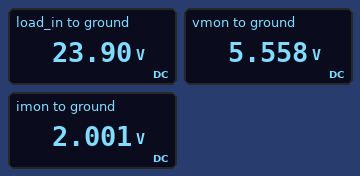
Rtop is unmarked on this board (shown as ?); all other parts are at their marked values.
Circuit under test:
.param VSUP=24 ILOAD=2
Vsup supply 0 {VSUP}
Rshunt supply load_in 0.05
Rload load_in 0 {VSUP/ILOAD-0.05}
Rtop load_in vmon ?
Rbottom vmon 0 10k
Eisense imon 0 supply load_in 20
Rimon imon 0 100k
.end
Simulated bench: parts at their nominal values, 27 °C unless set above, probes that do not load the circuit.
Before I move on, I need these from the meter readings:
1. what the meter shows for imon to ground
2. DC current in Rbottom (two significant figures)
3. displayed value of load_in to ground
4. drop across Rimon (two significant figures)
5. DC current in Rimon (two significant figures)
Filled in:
2.001 V
560 µA
23.90 V
2.0 V
20 µA
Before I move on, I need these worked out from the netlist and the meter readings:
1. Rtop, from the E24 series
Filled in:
33 kΩ
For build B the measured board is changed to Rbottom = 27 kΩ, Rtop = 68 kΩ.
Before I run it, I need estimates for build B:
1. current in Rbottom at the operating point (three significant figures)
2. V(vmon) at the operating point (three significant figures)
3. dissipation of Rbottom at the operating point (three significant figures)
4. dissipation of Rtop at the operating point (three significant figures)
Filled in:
252 µA
6.79 V
1.71 mW
4.30 mW
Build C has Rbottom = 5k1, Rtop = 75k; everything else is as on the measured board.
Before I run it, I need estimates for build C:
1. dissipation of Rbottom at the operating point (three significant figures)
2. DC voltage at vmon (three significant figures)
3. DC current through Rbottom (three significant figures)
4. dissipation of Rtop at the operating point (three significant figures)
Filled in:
454 µW
1.52 V
298 µA
6.68 mW
